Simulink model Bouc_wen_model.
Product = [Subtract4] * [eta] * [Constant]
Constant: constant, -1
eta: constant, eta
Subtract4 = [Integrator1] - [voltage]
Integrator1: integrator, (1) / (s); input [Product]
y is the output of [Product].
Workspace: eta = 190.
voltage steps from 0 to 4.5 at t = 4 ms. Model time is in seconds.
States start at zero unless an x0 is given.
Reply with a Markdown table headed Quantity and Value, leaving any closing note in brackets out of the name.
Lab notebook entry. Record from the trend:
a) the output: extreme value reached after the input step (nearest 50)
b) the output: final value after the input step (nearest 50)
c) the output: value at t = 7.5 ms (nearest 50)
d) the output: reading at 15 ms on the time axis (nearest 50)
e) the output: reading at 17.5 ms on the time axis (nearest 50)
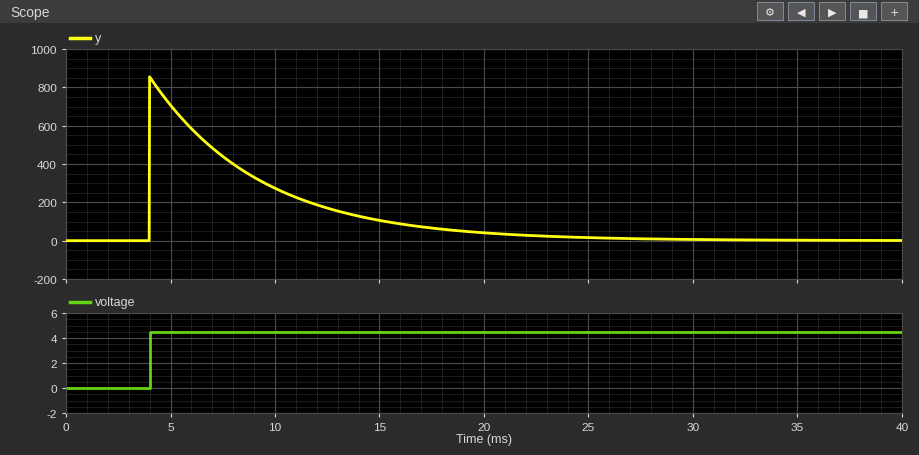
| Quantity | Value |
|---|---|
| the output: extreme value reached after the input step | 850 |
| the output: final value after the input step | 0 |
| the output: value at t = 7.5 ms | 450 |
| the output: reading at 15 ms on the time axis | 100 |
| the output: reading at 17.5 ms on the time axis | 50 |
